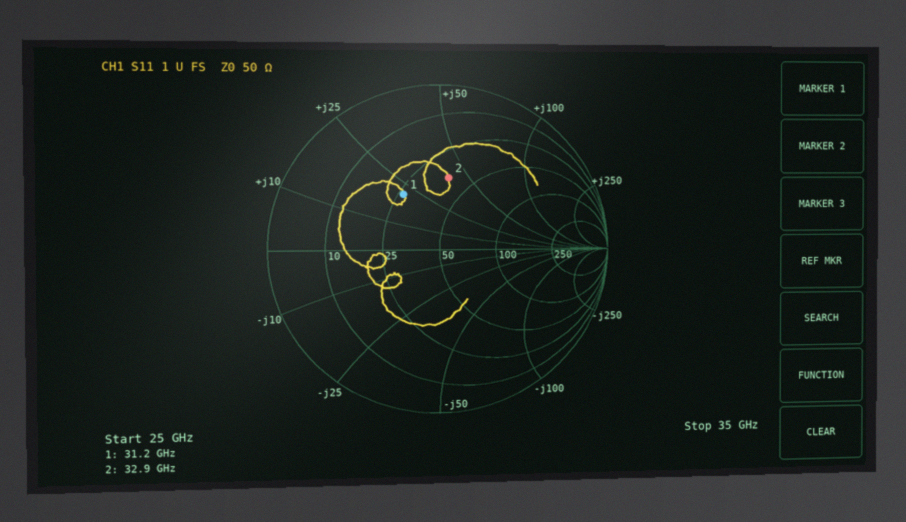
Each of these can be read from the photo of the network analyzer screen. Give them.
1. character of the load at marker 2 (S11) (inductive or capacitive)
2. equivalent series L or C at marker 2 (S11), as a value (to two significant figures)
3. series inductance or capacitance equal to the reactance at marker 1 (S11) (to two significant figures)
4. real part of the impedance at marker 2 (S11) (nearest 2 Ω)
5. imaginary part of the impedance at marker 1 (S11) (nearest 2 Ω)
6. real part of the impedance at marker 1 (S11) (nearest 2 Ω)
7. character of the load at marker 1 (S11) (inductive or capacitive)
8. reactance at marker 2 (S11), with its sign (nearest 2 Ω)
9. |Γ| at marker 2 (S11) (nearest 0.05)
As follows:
inductive
190 pH
110 pH
38 Ω
+22 Ω
26 Ω
inductive
+40 Ω
0.45
